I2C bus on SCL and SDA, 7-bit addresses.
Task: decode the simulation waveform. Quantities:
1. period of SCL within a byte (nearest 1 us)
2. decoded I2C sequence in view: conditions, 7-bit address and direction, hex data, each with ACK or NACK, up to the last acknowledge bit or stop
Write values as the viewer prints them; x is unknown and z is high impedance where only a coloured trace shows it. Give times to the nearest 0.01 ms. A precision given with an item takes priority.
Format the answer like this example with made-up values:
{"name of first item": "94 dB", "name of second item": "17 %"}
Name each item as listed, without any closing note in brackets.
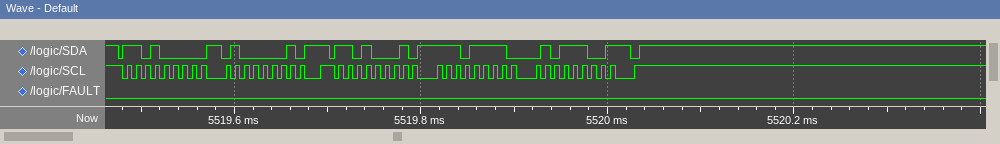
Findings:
{"period of SCL within a byte": "10 us", "decoded I2C sequence in view: conditions, 7-bit address and direction, hex data, each with ACK or NACK, up to the last acknowledge bit or stop": "start, address 68 write ACK, 41 ACK, repeated start, address 68 read ACK, EF ACK, 5C NACK, stop"}
